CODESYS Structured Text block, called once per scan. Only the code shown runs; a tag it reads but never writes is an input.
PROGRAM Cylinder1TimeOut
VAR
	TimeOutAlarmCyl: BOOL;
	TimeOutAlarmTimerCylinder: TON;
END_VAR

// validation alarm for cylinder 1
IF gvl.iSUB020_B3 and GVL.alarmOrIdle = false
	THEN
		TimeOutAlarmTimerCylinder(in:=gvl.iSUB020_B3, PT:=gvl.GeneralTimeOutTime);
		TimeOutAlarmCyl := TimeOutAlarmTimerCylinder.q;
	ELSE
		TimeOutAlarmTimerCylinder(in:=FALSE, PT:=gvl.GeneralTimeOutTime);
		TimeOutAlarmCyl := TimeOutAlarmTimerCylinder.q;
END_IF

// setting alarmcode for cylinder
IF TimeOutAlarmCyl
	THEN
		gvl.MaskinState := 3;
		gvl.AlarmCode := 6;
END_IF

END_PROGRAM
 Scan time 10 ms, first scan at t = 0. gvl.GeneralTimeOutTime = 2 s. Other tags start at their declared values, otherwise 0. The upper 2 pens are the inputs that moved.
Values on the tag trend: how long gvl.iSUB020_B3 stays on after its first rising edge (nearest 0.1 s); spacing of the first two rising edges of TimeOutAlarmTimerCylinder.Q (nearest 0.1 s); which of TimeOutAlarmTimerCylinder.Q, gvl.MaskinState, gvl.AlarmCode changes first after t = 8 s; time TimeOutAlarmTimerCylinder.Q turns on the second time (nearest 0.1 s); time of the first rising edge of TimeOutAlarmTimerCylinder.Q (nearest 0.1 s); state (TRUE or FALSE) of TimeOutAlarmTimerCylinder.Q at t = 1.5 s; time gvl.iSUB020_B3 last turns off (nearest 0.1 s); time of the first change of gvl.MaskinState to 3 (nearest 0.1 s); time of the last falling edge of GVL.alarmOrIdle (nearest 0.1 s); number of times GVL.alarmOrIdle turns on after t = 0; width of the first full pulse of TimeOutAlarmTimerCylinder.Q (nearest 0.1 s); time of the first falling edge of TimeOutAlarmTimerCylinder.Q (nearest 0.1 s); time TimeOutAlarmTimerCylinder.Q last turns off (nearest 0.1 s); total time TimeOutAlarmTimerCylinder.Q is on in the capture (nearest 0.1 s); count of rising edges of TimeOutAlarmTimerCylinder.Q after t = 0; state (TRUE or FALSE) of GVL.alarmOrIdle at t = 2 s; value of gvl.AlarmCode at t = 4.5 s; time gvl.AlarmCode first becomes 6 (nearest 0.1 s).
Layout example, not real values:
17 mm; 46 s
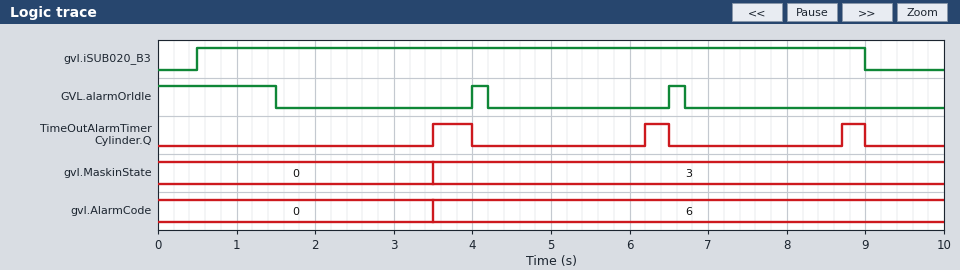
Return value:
8.5 s; 2.7 s; TimeOutAlarmTimerCylinder.Q; 6.2 s; 3.5 s; FALSE; 9.0 s; 3.5 s; 6.7 s; 2; 0.5 s; 4.0 s; 9.0 s; 1.1 s; 3; FALSE; 6; 3.5 s
